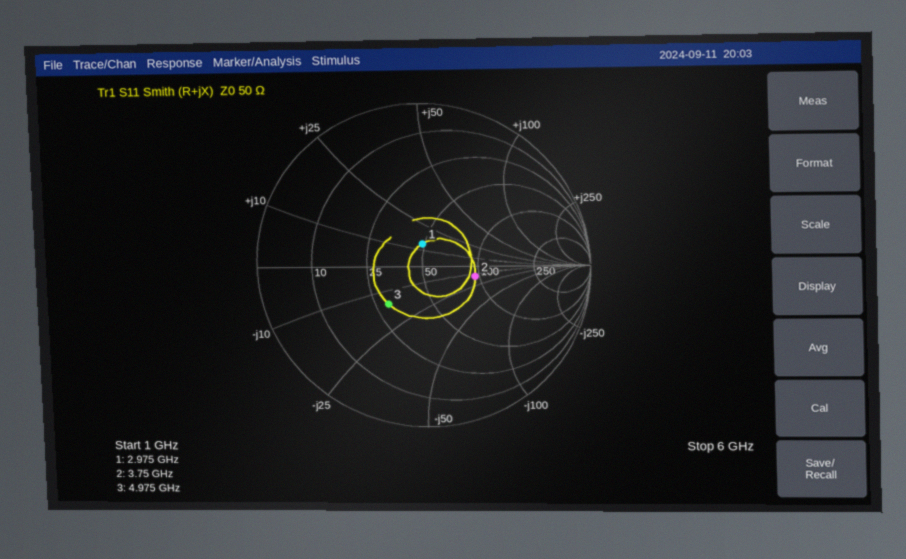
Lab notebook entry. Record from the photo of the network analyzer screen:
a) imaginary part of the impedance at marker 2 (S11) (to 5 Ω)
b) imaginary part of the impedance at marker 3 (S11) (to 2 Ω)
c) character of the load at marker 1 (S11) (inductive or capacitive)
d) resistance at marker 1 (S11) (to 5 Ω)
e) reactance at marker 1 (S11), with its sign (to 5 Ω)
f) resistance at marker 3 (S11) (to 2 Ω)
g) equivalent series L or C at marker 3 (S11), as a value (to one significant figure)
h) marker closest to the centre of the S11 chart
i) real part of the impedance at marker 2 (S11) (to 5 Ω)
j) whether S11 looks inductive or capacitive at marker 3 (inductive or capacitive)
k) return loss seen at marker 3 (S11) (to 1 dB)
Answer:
-15 Ω
-16 Ω
inductive
50 Ω
+15 Ω
30 Ω
2 pF
marker 1
95 Ω
capacitive
10 dB
